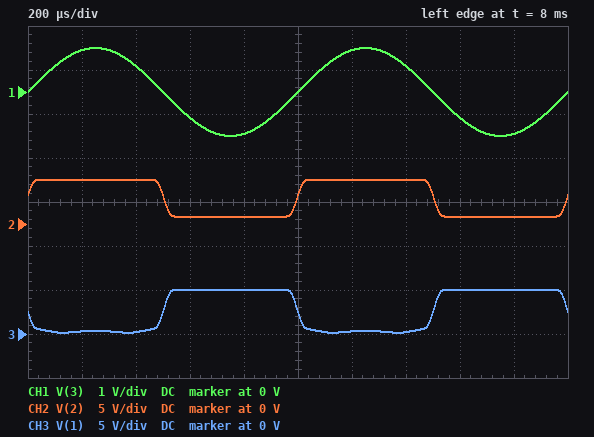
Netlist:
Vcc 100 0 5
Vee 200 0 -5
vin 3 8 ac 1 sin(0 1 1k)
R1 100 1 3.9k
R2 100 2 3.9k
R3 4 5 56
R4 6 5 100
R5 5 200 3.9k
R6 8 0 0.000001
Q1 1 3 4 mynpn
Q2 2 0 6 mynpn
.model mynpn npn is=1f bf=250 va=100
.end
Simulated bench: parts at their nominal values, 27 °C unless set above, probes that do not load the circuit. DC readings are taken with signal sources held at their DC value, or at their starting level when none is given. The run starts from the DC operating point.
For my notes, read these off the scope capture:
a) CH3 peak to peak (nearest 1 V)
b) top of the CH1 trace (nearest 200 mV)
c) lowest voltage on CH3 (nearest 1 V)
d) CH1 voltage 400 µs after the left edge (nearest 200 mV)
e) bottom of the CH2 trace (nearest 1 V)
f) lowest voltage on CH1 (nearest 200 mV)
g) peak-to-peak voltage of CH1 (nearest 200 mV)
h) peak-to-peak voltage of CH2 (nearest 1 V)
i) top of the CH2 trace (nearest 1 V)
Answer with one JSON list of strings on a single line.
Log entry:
["5 V", "1.0 V", "0 V", "600 mV", "1 V", "-1.0 V", "2.0 V", "4 V", "5 V"]
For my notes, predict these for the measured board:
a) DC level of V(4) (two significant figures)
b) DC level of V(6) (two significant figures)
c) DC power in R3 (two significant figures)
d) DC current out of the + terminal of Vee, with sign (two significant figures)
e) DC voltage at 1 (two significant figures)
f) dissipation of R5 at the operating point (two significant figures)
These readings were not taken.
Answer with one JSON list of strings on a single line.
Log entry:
["-700 mV", "-690 mV", "23 µW", "-1.1 mA", "2.5 V", "4.7 mW"]
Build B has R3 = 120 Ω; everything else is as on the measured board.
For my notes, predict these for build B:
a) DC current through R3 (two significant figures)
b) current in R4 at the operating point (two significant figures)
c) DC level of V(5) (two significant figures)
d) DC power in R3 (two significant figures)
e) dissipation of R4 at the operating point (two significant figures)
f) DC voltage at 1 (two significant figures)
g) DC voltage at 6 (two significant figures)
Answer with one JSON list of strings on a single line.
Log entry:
["510 µA", "580 µA", "-760 mV", "31 µW", "33 µW", "3.0 V", "-700 mV"]
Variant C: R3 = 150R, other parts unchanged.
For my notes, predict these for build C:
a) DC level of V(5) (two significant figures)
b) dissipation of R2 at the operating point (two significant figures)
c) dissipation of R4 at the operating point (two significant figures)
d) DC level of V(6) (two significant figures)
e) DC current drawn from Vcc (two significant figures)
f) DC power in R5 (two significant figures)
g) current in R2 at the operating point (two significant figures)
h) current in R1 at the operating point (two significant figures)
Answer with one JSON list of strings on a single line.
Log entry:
["-760 mV", "1.5 mW", "39 µW", "-700 mV", "1.1 mA", "4.6 mW", "620 µA", "460 µA"]
